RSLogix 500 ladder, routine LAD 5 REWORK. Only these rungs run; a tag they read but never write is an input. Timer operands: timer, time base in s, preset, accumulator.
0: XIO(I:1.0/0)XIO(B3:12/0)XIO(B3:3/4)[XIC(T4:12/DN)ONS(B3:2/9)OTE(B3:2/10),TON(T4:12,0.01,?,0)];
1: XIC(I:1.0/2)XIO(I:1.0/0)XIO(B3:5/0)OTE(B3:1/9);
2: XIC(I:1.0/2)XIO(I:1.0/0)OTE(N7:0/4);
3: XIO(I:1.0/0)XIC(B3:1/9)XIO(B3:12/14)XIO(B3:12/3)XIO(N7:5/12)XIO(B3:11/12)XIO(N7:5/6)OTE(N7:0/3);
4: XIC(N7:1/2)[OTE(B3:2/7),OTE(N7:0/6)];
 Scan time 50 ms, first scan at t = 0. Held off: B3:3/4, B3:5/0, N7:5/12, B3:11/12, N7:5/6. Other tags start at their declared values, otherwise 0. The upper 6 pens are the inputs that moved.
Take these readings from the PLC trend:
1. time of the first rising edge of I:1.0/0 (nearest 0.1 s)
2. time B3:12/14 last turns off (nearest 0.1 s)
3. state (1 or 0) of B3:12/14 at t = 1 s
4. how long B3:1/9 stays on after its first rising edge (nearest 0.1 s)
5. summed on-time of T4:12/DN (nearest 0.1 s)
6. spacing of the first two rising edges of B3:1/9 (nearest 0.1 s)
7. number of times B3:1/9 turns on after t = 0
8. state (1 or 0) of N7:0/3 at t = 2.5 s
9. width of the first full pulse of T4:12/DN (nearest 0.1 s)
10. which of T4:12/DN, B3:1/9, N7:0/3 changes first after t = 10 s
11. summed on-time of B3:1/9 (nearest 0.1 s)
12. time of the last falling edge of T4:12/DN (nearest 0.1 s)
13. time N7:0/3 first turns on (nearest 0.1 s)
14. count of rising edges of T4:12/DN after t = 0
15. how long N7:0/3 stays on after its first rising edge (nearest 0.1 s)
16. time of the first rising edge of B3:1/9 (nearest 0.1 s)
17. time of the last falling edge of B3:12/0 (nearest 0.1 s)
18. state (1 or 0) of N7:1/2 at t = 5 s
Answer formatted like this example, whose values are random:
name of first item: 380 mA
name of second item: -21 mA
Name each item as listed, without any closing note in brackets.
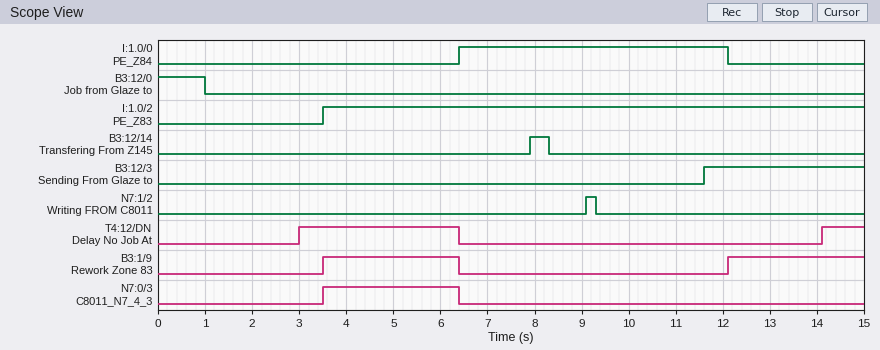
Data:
time of the first rising edge of I:1.0/0: 6.4 s
time B3:12/14 last turns off: 8.3 s
state (1 or 0) of B3:12/14 at t = 1 s: 0
how long B3:1/9 stays on after its first rising edge: 2.9 s
summed on-time of T4:12/DN: 4.3 s
spacing of the first two rising edges of B3:1/9: 8.6 s
number of times B3:1/9 turns on after t = 0: 2
state (1 or 0) of N7:0/3 at t = 2.5 s: 0
width of the first full pulse of T4:12/DN: 3.4 s
which of T4:12/DN, B3:1/9, N7:0/3 changes first after t = 10 s: B3:1/9
summed on-time of B3:1/9: 5.8 s
time of the last falling edge of T4:12/DN: 6.4 s
time N7:0/3 first turns on: 3.5 s
count of rising edges of T4:12/DN after t = 0: 2
how long N7:0/3 stays on after its first rising edge: 2.9 s
time of the first rising edge of B3:1/9: 3.5 s
time of the last falling edge of B3:12/0: 1.0 s
state (1 or 0) of N7:1/2 at t = 5 s: 0
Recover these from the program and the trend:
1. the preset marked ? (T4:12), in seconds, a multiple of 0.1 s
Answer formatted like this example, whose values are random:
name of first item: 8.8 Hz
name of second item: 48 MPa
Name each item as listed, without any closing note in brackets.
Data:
the preset marked ? (T4:12), in seconds, a multiple of 0.1 s: 2.0 s
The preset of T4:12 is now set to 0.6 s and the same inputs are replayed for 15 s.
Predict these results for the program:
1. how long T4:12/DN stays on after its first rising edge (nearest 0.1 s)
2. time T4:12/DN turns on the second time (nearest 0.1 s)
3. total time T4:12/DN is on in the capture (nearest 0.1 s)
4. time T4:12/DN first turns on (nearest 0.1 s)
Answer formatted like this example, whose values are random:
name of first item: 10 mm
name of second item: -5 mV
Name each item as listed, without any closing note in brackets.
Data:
how long T4:12/DN stays on after its first rising edge: 4.8 s
time T4:12/DN turns on the second time: 12.7 s
total time T4:12/DN is on in the capture: 7.1 s
time T4:12/DN first turns on: 1.6 s
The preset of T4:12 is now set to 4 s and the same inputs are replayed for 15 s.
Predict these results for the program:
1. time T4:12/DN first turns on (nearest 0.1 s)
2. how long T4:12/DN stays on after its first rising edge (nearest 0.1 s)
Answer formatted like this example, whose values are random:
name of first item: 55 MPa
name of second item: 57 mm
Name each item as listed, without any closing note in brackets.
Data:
time T4:12/DN first turns on: 5.0 s
how long T4:12/DN stays on after its first rising edge: 1.4 s
